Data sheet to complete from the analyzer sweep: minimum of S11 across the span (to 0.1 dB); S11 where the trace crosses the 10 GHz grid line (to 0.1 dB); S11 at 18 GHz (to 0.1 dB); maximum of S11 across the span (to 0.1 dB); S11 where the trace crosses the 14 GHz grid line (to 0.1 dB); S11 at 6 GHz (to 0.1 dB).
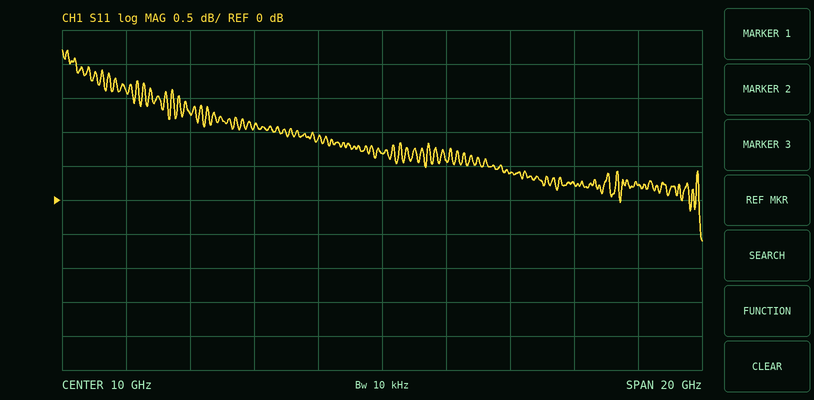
-0.6 dB
0.7 dB
0.2 dB
2.2 dB
0.4 dB
1.1 dB
